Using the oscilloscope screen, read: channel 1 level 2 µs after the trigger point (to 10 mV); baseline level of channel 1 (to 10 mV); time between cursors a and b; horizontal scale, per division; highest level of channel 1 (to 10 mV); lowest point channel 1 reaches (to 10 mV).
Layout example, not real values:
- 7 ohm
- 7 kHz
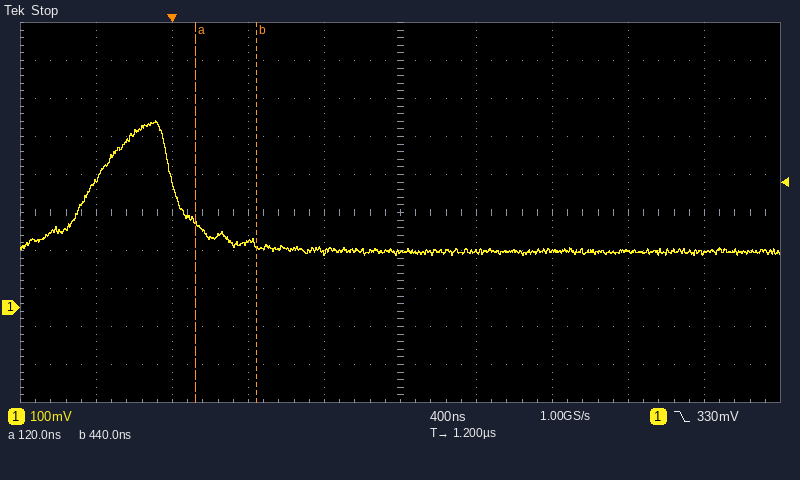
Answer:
- 150 mV
- 150 mV
- 320 ns
- 400 ns
- 490 mV
- 140 mV
